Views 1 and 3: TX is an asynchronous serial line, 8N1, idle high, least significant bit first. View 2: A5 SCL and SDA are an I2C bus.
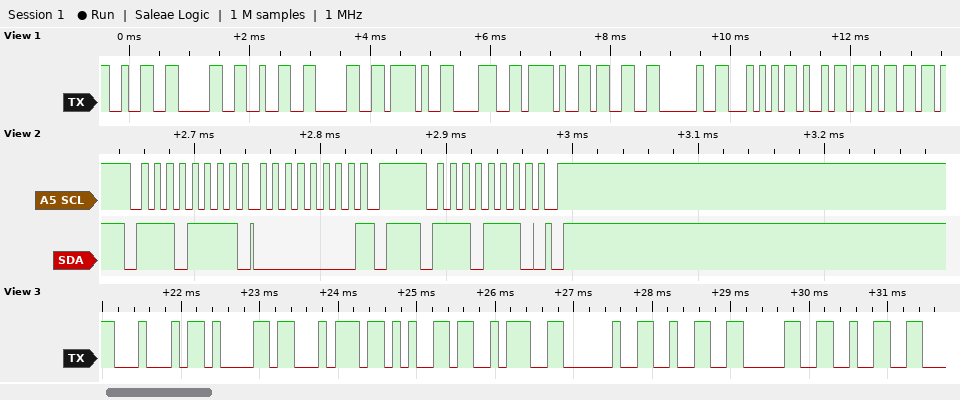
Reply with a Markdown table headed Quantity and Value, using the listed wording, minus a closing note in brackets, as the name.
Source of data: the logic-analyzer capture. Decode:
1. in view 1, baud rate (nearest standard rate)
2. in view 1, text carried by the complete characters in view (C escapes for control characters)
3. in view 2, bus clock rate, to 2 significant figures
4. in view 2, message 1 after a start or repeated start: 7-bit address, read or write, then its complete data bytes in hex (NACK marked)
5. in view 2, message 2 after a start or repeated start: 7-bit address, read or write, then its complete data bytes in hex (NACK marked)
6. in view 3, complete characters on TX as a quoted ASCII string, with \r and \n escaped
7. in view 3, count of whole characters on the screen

| Quantity | Value |
|---|---|
| in view 1, baud rate | 9600 baud |
| in view 1, text carried by the complete characters in view | "2020/8/3 Tim" |
| in view 2, bus clock rate, to 2 significant figures | 100 kHz |
| in view 2, message 1 after a start or repeated start: 7-bit address, read or write, then its complete data bytes in hex | 0x77 read: 00 NACK |
| in view 2, message 2 after a start or repeated start: 7-bit address, read or write, then its complete data bytes in hex | 0x77 write |
| in view 3, complete characters on TX as a quoted ASCII string, with \r and \n escaped | "Date: 202" |
| in view 3, count of whole characters on the screen | 9 |
